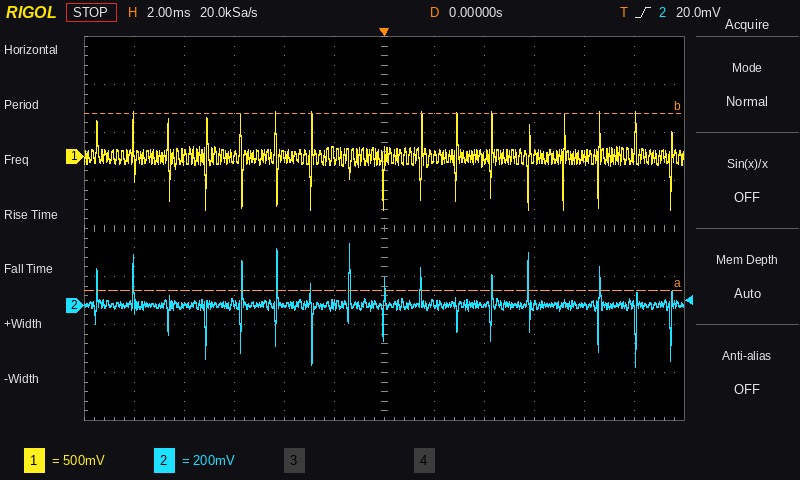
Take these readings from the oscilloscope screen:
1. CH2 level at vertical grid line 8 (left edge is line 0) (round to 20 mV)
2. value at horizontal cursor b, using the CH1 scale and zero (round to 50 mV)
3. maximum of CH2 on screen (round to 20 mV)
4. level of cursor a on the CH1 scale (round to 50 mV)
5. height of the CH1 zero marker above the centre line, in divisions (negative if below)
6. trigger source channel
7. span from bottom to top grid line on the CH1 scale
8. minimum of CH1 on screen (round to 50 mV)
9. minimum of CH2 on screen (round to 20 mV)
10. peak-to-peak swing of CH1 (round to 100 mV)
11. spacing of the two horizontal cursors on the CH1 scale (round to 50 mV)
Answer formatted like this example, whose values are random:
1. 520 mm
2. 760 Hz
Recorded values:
1. 0 mV
2. 450 mV
3. 260 mV
4. -1.40 V
5. +1.5 div
6. CH2
7. 4 V
8. -550 mV
9. -260 mV
10. 1.00 V
11. 1.85 V
